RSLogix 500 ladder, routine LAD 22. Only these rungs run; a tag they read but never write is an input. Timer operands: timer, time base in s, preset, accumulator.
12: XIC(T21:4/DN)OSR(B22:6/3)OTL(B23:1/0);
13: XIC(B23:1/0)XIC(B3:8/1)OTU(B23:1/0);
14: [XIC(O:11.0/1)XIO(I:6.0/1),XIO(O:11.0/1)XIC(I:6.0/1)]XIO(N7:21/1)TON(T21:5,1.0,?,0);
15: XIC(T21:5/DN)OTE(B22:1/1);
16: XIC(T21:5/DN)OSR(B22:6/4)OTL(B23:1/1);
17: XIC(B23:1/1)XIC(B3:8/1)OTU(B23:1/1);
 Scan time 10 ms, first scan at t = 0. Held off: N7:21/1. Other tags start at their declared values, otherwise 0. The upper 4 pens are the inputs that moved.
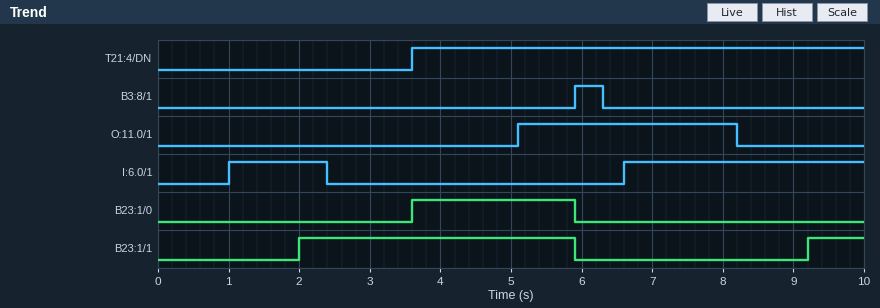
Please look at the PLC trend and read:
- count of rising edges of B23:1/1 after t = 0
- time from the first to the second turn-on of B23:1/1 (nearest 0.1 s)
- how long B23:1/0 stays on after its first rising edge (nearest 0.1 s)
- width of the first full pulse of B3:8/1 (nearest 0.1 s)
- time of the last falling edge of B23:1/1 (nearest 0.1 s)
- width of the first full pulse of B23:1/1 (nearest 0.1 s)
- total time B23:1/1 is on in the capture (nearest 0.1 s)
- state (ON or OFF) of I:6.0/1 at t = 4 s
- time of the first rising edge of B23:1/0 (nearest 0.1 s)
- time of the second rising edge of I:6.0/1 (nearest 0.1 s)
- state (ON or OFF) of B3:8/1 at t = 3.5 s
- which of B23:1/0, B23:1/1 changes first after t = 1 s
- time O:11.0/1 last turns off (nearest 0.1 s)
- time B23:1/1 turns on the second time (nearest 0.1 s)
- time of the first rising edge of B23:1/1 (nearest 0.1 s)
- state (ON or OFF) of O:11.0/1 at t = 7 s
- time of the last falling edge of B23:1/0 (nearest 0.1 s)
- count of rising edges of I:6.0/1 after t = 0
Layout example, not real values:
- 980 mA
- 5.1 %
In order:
- 2
- 7.2 s
- 2.3 s
- 0.4 s
- 5.9 s
- 3.9 s
- 4.7 s
- OFF
- 3.6 s
- 6.6 s
- OFF
- B23:1/1
- 8.2 s
- 9.2 s
- 2.0 s
- ON
- 5.9 s
- 2
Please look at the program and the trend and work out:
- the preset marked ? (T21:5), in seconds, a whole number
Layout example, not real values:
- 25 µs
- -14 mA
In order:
- 1 s
